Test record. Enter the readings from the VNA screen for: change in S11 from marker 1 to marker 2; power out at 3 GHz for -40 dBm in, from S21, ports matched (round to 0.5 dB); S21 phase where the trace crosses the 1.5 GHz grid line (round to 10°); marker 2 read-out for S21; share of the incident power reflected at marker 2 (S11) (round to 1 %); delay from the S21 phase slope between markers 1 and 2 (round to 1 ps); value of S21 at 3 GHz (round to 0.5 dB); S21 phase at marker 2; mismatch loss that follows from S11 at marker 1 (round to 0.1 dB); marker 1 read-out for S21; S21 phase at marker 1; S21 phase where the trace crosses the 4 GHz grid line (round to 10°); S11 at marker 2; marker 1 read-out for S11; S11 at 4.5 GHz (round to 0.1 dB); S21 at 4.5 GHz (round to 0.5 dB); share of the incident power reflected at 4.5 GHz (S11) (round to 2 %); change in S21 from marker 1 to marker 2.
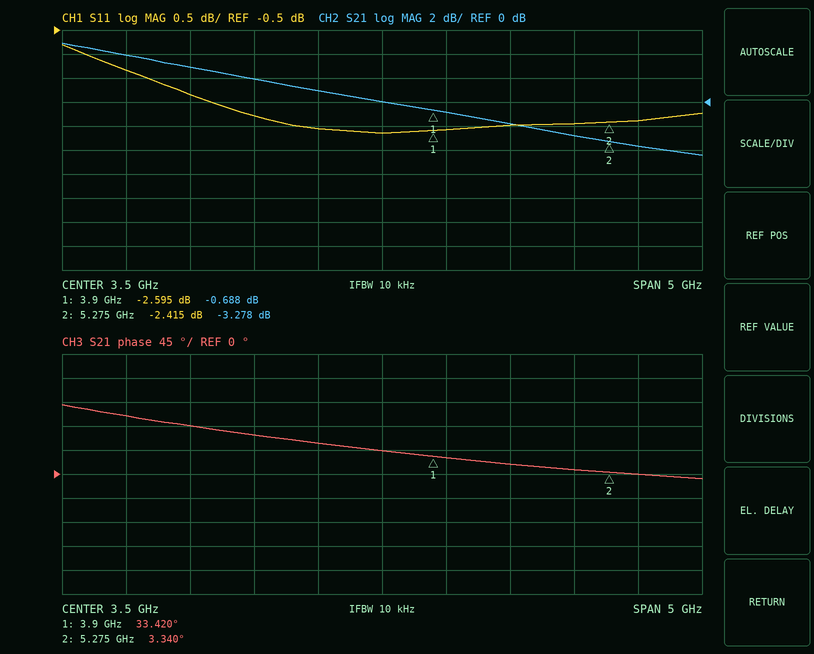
0.180 dB
-39.0 dBm
110°
-3.278 dB
57 %
61 ps
1.0 dB
3.340°
3.5 dB
-0.688 dB
33.420°
30°
-2.415 dB
-2.595 dB
-2.5 dB
-2.0 dB
56 %
-2.590 dB
